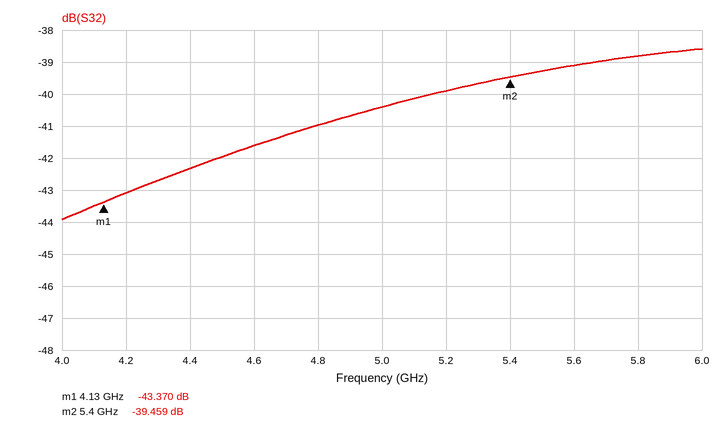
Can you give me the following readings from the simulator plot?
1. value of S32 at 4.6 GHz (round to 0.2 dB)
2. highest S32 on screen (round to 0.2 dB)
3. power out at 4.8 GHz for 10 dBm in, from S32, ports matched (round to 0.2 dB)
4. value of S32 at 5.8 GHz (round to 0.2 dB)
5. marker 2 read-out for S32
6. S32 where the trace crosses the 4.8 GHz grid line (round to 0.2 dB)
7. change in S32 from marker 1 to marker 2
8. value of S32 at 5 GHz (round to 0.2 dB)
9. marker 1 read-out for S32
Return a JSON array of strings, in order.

["-41.6 dB", "-38.6 dB", "-31.0 dBm", "-38.8 dB", "-39.459 dB", "-41.0 dB", "3.911 dB", "-40.4 dB", "-43.370 dB"]
